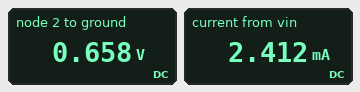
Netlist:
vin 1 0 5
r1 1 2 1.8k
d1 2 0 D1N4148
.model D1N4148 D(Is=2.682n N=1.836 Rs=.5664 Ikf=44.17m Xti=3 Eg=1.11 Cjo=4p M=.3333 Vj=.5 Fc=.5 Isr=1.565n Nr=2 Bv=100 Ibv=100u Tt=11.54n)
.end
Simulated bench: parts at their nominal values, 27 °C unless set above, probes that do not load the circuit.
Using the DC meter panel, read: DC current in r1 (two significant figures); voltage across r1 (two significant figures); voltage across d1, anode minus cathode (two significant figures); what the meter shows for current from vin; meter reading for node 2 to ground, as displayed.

2.4 mA
4.3 V
660 mV
2.412 mA
0.658 V
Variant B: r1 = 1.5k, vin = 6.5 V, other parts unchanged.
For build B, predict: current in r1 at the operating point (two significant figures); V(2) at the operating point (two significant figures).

3.9 mA
680 mV
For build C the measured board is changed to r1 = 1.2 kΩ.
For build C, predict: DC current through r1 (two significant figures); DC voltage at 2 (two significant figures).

3.6 mA
680 mV
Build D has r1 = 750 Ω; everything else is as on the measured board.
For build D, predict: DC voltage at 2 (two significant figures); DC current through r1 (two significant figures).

710 mV
5.7 mA
